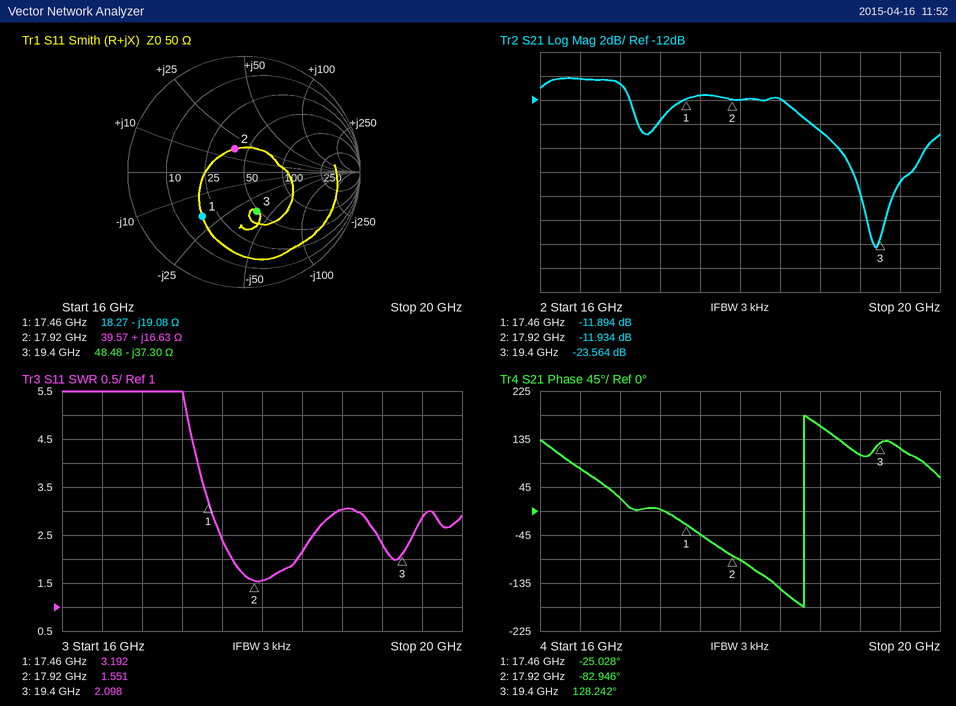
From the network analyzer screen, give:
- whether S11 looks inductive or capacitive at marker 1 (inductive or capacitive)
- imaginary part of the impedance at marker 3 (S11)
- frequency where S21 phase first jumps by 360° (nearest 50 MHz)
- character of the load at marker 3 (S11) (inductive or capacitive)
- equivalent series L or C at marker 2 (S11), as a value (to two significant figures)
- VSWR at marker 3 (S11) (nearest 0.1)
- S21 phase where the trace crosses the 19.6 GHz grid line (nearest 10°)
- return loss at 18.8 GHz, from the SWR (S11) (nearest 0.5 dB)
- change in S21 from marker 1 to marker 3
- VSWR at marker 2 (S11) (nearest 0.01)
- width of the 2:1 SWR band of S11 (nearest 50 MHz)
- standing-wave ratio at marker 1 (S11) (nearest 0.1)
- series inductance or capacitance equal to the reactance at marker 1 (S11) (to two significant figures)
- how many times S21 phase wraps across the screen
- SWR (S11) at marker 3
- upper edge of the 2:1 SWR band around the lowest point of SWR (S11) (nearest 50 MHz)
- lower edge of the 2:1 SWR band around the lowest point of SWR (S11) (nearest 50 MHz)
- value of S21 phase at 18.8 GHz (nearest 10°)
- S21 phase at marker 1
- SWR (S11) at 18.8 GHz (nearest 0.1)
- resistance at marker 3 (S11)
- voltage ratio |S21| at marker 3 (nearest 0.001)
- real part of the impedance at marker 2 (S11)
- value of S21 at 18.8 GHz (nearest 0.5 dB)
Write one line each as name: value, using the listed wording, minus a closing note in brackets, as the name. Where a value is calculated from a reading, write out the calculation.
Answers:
whether S11 looks inductive or capacitive at marker 1: capacitive
imaginary part of the impedance at marker 3: -37.30 Ω
frequency where S21 phase first jumps by 360°: 18.65 GHz
character of the load at marker 3 (S11): capacitive
equivalent series L or C at marker 2 (S11), as a value: L = 16.63 Ω/(2π × 17.92 GHz) ≈ 148 pH, so 150 pH to two significant figures
VSWR at marker 3 (S11): 2.1
S21 phase where the trace crosses the 19.6 GHz grid line: 120°
return loss at 18.8 GHz, from the SWR (S11): −20 log10((3 − 1)/(3 + 1)) ≈ 6.0 dB
change in S21 from marker 1 to marker 3: -23.564 − (-11.894) = -11.670 dB
VSWR at marker 2 (S11): 1.55
width of the 2:1 SWR band of S11: 18.35 GHz − 17.70 GHz = 650 MHz
standing-wave ratio at marker 1 (S11): 3.2
series inductance or capacitance equal to the reactance at marker 1 (S11): C = 1/(2π × 17.46 GHz × 19.08 Ω) ≈ 478 fF, so 480 fF to two significant figures
how many times S21 phase wraps across the screen: 1
SWR (S11) at marker 3: 2.098
upper edge of the 2:1 SWR band around the lowest point of SWR (S11): 18.35 GHz
lower edge of the 2:1 SWR band around the lowest point of SWR (S11): 17.70 GHz
value of S21 phase at 18.8 GHz: 160°
S21 phase at marker 1: -25.028°
SWR (S11) at 18.8 GHz: 3.0
resistance at marker 3: 48.48 Ω
voltage ratio |S21| at marker 3: 10^(-23.564/20) ≈ 0.066
real part of the impedance at marker 2: 39.57 Ω
value of S21 at 18.8 GHz: -14.5 dB
